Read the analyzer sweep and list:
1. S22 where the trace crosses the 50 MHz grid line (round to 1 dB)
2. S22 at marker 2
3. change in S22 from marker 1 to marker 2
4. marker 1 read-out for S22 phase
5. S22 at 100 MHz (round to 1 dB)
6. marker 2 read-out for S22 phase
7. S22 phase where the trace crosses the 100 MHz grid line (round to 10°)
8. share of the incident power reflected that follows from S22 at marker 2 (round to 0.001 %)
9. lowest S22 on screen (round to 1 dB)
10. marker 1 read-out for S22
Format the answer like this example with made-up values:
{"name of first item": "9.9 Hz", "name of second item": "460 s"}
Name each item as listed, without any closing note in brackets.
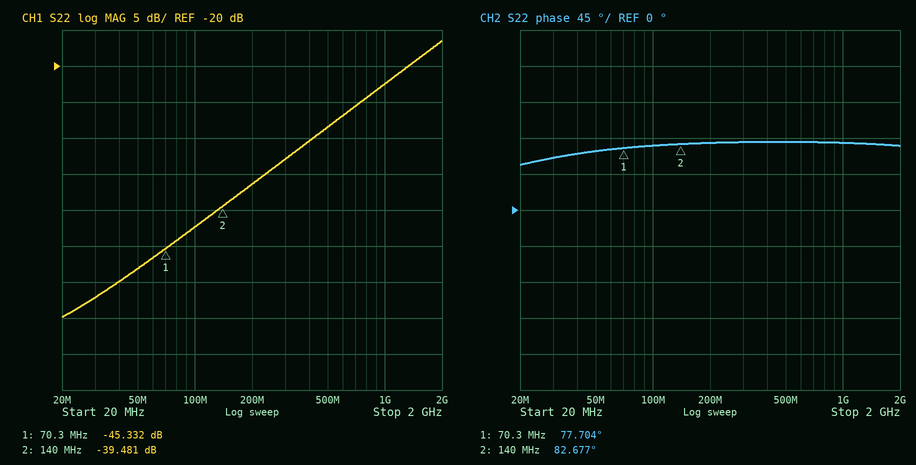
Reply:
{"S22 where the trace crosses the 50 MHz grid line": "-48 dB", "S22 at marker 2": "-39.481 dB", "change in S22 from marker 1 to marker 2": "5.851 dB", "marker 1 read-out for S22 phase": "77.704°", "S22 at 100 MHz": "-42 dB", "marker 2 read-out for S22 phase": "82.677°", "S22 phase where the trace crosses the 100 MHz grid line": "80°", "share of the incident power reflected that follows from S22 at marker 2": "0.011 %", "lowest S22 on screen": "-55 dB", "marker 1 read-out for S22": "-45.332 dB"}
